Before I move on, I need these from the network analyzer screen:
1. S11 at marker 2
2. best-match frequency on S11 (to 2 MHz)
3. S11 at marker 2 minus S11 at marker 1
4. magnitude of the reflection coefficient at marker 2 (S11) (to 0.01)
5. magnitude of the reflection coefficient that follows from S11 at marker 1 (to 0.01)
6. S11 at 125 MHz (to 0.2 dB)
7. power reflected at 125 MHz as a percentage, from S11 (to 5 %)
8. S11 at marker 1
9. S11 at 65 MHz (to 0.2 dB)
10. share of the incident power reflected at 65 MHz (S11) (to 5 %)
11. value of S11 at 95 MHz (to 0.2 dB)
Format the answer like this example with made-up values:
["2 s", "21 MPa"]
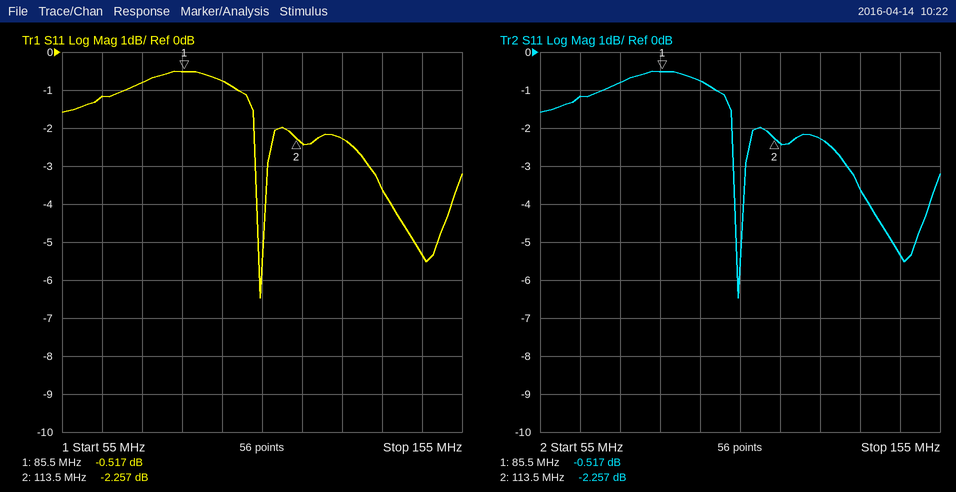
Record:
["-2.257 dB", "104 MHz", "-1.740 dB", "0.77", "0.94", "-2.2 dB", "60 %", "-0.517 dB", "-1.2 dB", "75 %", "-0.8 dB"]
